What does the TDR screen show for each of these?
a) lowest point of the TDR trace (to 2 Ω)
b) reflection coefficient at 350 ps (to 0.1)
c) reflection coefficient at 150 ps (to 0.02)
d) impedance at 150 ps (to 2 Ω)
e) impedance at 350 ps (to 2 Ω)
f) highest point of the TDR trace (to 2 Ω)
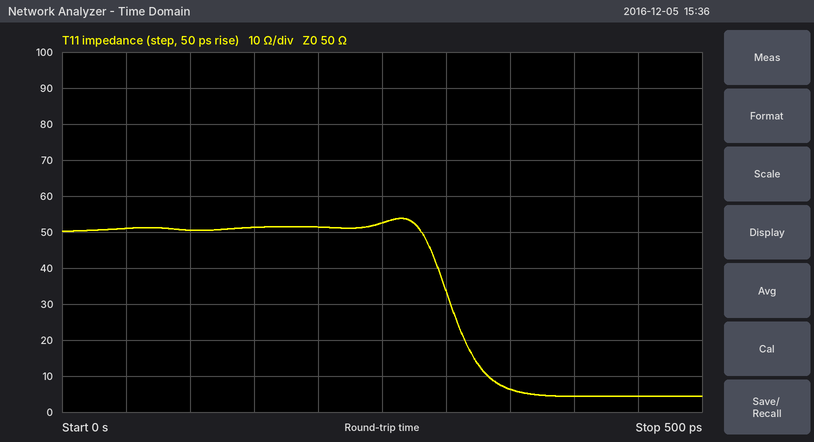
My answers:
4 Ω
-0.8
+0.02
52 Ω
6 Ω
54 Ω
